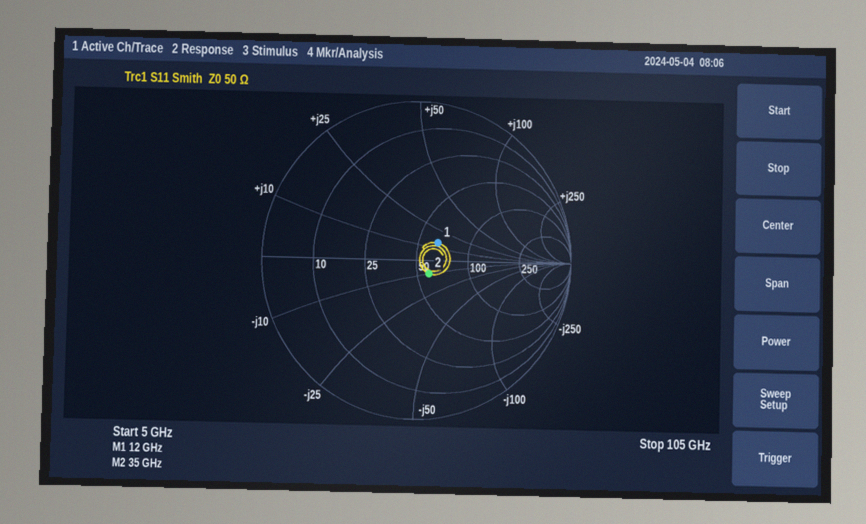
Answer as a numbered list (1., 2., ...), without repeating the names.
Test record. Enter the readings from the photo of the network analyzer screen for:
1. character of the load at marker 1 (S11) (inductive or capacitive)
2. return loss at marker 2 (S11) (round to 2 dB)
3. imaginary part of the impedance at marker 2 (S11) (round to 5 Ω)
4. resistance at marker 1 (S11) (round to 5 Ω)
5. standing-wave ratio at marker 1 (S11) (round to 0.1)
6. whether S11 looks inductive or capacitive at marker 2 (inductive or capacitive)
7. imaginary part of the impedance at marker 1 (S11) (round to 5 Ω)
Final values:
1. inductive
2. 18 dB
3. -10 Ω
4. 65 Ω
5. 1.4
6. capacitive
7. +15 Ω
